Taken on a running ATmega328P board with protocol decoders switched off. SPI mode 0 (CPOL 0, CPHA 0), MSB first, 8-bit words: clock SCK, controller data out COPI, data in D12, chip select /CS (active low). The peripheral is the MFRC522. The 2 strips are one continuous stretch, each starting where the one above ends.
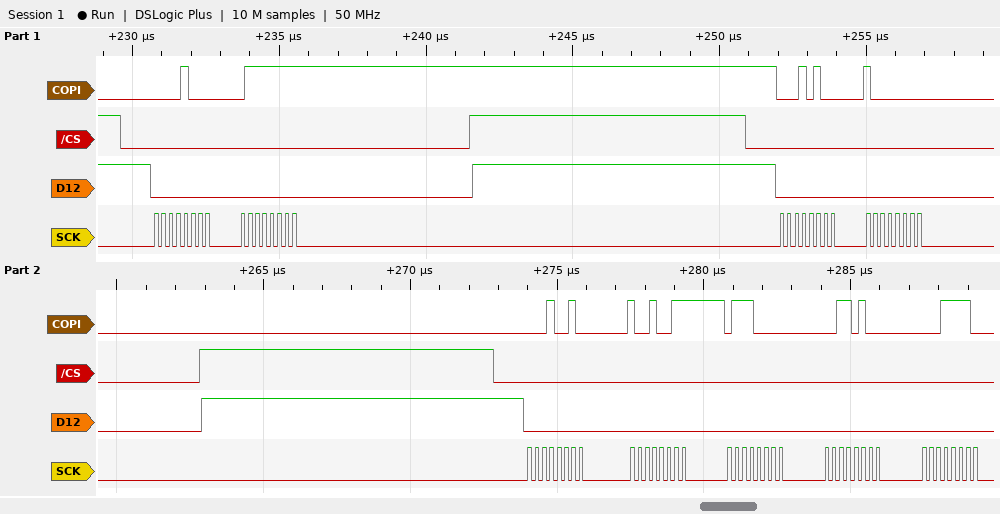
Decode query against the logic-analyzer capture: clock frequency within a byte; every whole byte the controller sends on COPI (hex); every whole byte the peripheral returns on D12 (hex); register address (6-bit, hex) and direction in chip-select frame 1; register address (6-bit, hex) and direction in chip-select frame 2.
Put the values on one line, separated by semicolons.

4 MHz; 08 7F 14 80 12 93 70 34 1E; 00 00 00 00 00 00 00 00 00; 0x04 write; 0x0A write
